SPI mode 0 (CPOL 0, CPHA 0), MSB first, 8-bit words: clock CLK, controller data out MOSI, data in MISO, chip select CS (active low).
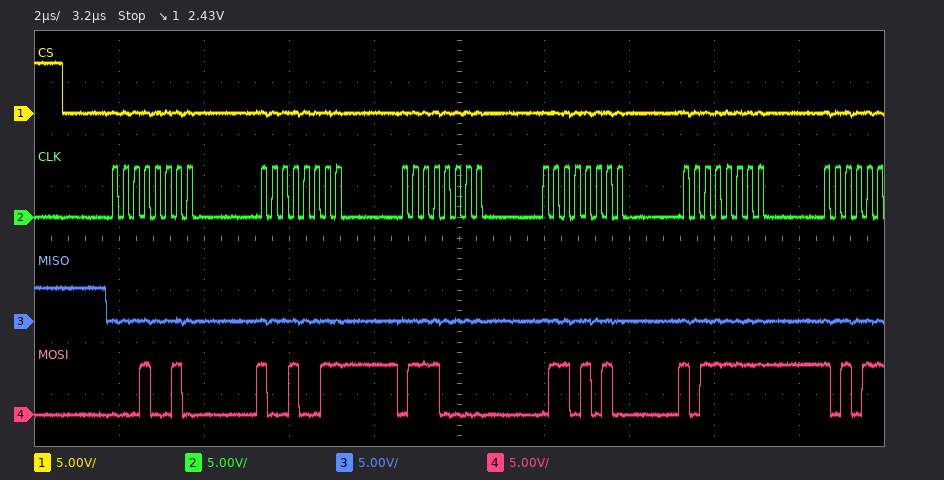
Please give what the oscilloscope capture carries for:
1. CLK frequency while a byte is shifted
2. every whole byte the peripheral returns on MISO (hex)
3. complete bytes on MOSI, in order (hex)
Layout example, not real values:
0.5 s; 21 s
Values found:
4 MHz; 00 00 00 00 00; 12 93 70 6A BF
